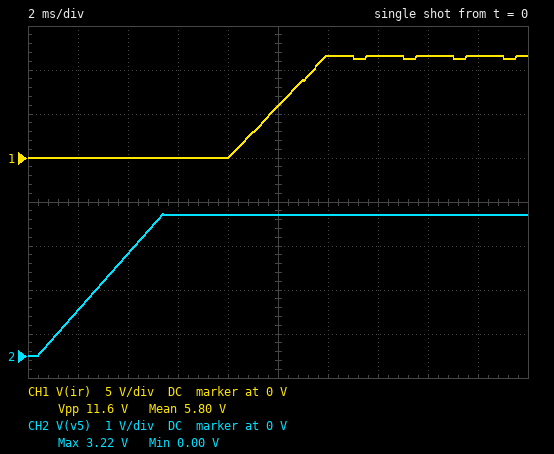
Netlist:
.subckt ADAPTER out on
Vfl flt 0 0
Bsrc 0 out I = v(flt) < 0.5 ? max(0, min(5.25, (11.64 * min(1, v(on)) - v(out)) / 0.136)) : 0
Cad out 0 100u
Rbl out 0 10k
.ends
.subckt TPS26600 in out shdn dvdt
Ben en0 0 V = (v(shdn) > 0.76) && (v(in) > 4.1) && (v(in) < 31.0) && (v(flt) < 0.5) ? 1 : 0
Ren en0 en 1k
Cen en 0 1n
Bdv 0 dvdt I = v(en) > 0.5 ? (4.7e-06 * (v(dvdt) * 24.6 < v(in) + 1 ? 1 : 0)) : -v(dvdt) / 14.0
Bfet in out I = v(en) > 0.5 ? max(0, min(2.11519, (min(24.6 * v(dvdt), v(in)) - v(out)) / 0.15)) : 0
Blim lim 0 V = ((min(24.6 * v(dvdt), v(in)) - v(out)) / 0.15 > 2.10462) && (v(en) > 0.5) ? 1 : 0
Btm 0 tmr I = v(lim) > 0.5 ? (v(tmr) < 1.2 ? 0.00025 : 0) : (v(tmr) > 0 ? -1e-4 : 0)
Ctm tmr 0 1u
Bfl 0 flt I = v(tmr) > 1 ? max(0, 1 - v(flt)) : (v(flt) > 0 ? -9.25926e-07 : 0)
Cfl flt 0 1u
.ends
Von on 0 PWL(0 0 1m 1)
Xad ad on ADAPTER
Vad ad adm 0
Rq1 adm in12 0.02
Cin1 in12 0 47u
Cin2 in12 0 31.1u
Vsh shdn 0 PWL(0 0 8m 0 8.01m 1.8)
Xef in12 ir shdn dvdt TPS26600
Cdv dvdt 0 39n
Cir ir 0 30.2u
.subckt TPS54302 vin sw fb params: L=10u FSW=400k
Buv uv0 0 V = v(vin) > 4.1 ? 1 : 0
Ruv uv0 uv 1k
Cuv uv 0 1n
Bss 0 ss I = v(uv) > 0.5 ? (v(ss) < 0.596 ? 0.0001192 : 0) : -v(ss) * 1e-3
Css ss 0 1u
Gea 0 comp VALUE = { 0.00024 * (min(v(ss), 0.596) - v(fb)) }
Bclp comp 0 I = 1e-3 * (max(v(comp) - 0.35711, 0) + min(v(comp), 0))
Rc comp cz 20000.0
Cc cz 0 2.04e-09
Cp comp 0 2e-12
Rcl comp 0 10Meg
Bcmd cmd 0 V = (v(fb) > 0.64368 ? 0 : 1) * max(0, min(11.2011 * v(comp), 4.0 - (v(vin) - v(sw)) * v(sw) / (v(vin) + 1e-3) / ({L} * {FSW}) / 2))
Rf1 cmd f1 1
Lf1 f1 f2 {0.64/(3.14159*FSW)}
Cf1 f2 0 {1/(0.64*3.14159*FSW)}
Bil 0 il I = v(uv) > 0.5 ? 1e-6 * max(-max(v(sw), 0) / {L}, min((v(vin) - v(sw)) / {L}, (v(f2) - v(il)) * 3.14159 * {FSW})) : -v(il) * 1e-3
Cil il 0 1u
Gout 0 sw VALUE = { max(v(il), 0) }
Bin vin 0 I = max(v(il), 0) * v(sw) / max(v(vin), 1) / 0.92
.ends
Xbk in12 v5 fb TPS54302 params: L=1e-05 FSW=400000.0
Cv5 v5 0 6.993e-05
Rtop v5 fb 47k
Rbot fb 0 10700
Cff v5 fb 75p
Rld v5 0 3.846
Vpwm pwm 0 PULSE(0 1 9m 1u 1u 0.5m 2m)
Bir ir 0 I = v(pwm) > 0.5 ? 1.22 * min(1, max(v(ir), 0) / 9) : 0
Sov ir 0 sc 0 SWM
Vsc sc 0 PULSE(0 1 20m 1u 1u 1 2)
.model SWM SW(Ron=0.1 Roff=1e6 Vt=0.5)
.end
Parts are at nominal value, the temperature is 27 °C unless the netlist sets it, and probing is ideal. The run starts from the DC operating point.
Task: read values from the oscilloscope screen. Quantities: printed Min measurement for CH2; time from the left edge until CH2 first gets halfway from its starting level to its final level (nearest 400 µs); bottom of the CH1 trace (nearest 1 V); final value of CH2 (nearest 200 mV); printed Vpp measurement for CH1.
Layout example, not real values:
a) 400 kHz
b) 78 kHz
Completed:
a) 0.00 V
b) 2.8 ms
c) 0 V
d) 3.2 V
e) 11.6 V
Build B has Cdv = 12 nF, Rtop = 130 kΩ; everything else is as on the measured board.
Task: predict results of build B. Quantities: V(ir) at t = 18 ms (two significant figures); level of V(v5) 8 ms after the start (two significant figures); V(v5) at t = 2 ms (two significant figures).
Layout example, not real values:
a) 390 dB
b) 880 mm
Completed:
a) 11 V
b) 7.8 V
c) 2.5 V
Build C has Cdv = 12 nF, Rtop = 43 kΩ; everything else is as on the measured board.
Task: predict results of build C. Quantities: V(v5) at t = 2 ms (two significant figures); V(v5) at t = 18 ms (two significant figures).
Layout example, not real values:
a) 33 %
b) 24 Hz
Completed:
a) 970 mV
b) 3.0 V
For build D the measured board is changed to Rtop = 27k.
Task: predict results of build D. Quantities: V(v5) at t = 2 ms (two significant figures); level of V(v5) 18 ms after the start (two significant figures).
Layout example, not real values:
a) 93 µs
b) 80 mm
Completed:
a) 680 mV
b) 2.1 V
